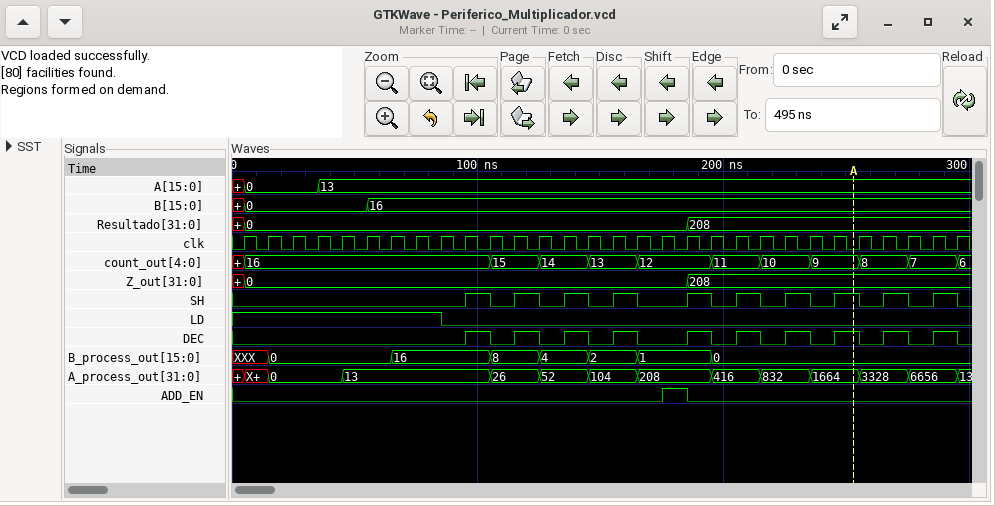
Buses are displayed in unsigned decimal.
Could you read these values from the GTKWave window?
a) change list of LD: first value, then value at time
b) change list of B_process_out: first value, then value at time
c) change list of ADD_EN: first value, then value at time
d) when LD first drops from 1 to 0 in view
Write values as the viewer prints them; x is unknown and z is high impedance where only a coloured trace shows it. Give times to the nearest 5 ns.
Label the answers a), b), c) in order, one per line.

a) 1, 0 at 85 ns
b) XXX, 0 at 15 ns, 16 at 65 ns, 8 at 105 ns, 4 at 125 ns, 2 at 145 ns, 1 at 165 ns, 0 at 195 ns
c) 0, 1 at 175 ns, 0 at 185 ns
d) 85 ns
